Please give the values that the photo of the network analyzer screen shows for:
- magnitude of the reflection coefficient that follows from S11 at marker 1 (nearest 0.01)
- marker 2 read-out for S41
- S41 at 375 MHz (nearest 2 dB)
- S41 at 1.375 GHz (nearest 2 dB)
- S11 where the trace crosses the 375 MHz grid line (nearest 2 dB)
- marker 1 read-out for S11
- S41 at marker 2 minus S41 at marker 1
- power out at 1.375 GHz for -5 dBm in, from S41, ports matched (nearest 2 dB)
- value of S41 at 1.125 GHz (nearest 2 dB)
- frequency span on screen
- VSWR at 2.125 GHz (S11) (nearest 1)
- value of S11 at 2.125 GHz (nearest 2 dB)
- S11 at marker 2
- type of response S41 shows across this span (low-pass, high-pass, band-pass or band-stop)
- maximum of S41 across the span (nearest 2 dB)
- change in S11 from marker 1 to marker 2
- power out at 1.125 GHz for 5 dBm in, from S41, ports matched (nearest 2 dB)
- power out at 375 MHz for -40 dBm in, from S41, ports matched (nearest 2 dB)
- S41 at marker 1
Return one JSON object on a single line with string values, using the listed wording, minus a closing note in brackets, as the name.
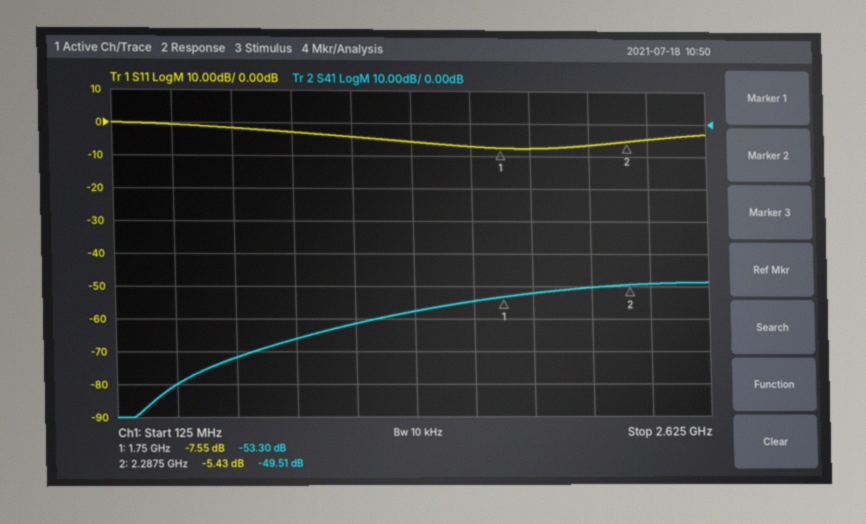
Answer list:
{"magnitude of the reflection coefficient that follows from S11 at marker 1": "0.42", "marker 2 read-out for S41": "-49.51 dB", "S41 at 375 MHz": "-80 dB", "S41 at 1.375 GHz": "-58 dB", "S11 where the trace crosses the 375 MHz grid line": "0 dB", "marker 1 read-out for S11": "-7.55 dB", "S41 at marker 2 minus S41 at marker 1": "3.79 dB", "power out at 1.375 GHz for -5 dBm in, from S41, ports matched": "-62 dBm", "value of S41 at 1.125 GHz": "-62 dB", "frequency span on screen": "2.5 GHz", "VSWR at 2.125 GHz (S11)": "3", "value of S11 at 2.125 GHz": "-6 dB", "S11 at marker 2": "-5.43 dB", "type of response S41 shows across this span": "high-pass", "maximum of S41 across the span": "-48 dB", "change in S11 from marker 1 to marker 2": "2.12 dB", "power out at 1.125 GHz for 5 dBm in, from S41, ports matched": "-56 dBm", "power out at 375 MHz for -40 dBm in, from S41, ports matched": "-120 dBm", "S41 at marker 1": "-53.30 dB"}
